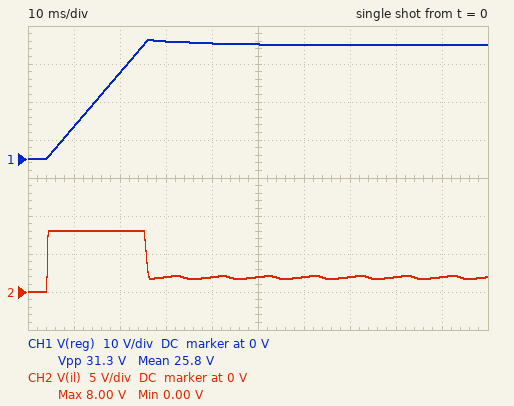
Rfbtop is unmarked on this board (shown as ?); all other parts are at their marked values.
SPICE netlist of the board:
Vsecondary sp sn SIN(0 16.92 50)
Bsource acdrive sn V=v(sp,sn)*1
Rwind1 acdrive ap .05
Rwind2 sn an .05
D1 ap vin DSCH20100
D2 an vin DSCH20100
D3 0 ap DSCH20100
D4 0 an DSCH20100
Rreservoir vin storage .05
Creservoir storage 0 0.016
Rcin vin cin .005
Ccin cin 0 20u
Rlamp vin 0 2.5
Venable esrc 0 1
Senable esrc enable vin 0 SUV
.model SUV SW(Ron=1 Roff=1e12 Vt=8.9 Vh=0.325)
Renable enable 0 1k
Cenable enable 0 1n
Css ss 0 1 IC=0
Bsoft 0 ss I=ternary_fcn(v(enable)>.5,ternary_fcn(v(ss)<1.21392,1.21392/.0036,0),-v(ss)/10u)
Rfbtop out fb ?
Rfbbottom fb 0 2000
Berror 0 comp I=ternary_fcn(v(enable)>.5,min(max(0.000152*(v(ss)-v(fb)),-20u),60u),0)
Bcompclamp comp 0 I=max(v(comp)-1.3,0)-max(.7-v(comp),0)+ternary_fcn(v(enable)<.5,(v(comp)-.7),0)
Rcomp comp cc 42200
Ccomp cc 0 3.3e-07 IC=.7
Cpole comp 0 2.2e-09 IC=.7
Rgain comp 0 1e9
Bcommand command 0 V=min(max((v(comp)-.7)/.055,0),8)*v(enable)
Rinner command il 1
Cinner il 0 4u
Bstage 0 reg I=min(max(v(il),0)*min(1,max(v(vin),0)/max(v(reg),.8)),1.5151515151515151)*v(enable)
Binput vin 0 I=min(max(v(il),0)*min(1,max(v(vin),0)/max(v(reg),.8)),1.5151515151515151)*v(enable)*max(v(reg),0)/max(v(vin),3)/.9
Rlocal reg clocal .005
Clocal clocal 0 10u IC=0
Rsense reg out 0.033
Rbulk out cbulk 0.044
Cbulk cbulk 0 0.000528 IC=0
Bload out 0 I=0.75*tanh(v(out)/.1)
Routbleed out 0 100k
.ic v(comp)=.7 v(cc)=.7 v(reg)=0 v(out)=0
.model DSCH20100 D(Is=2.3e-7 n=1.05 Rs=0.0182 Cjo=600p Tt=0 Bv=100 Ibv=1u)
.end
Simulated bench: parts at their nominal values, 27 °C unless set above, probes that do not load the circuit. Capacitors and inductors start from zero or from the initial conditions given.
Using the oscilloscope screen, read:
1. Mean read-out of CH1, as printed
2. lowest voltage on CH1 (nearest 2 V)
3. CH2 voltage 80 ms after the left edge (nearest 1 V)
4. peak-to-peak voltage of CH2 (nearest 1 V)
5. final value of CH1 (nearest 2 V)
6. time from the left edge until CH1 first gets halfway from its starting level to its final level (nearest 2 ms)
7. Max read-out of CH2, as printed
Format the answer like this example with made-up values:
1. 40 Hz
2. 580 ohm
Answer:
1. 25.8 V
2. 0 V
3. 2 V
4. 8 V
5. 30 V
6. 14 ms
7. 8.00 V
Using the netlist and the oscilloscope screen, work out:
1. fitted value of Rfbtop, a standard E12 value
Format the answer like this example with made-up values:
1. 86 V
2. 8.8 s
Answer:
1. 47 kΩ
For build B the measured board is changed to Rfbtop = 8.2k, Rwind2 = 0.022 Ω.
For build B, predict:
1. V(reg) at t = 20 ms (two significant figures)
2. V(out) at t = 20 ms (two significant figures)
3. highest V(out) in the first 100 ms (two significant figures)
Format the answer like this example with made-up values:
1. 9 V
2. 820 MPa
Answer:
1. 6.3 V
2. 6.2 V
3. 6.4 V
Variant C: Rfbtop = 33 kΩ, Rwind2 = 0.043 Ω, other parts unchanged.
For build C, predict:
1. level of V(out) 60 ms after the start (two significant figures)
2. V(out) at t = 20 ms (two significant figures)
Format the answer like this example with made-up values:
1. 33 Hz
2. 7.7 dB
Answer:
1. 21 V
2. 22 V
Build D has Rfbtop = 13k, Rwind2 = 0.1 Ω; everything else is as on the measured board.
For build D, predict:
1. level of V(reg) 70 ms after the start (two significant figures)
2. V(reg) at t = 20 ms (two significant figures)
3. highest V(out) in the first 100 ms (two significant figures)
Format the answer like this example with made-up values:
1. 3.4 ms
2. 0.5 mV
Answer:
1. 9.1 V
2. 9.2 V
3. 9.4 V
